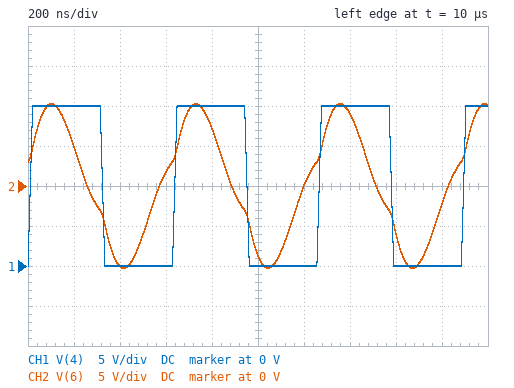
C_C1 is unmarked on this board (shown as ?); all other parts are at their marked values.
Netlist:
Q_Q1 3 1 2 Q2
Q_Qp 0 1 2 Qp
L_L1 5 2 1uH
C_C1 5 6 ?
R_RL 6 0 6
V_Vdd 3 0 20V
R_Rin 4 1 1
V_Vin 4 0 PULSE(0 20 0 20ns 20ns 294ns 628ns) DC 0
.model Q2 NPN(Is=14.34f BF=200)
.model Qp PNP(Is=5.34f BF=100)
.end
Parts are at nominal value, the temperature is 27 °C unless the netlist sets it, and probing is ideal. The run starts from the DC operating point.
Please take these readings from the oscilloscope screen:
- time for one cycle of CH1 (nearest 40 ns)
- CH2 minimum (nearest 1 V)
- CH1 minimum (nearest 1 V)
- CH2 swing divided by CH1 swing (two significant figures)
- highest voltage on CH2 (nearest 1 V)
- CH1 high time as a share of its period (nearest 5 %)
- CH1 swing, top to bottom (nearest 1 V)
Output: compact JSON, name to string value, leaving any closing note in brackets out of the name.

{"time for one cycle of CH1": "640 ns", "CH2 minimum": "-10 V", "CH1 minimum": "0 V", "CH2 swing divided by CH1 swing": "1.0", "highest voltage on CH2": "10 V", "CH1 high time as a share of its period": "50 %", "CH1 swing, top to bottom": "20 V"}
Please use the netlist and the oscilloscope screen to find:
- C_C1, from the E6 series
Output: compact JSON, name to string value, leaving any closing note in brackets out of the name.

{"C_C1, from the E6 series": "6.8 nF"}
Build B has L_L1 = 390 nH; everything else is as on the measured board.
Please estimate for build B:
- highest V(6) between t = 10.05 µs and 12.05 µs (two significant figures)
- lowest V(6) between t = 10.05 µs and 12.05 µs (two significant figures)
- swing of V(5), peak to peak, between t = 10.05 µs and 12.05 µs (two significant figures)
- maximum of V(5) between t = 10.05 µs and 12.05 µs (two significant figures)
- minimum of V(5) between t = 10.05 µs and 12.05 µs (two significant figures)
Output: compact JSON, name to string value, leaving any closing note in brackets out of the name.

{"highest V(6) between t = 10.05 µs and 12.05 µs": "9.2 V", "lowest V(6) between t = 10.05 µs and 12.05 µs": "-9.2 V", "swing of V(5), peak to peak, between t = 10.05 µs and 12.05 µs": "32 V", "maximum of V(5) between t = 10.05 µs and 12.05 µs": "26 V", "minimum of V(5) between t = 10.05 µs and 12.05 µs": "-6.2 V"}
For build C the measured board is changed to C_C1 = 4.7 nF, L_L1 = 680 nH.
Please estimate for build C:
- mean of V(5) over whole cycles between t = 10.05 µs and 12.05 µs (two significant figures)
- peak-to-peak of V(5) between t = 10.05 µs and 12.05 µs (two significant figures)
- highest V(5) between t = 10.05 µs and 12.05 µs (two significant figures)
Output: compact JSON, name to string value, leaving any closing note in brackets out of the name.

{"mean of V(5) over whole cycles between t = 10.05 µs and 12.05 µs": "10 V", "peak-to-peak of V(5) between t = 10.05 µs and 12.05 µs": "37 V", "highest V(5) between t = 10.05 µs and 12.05 µs": "28 V"}
